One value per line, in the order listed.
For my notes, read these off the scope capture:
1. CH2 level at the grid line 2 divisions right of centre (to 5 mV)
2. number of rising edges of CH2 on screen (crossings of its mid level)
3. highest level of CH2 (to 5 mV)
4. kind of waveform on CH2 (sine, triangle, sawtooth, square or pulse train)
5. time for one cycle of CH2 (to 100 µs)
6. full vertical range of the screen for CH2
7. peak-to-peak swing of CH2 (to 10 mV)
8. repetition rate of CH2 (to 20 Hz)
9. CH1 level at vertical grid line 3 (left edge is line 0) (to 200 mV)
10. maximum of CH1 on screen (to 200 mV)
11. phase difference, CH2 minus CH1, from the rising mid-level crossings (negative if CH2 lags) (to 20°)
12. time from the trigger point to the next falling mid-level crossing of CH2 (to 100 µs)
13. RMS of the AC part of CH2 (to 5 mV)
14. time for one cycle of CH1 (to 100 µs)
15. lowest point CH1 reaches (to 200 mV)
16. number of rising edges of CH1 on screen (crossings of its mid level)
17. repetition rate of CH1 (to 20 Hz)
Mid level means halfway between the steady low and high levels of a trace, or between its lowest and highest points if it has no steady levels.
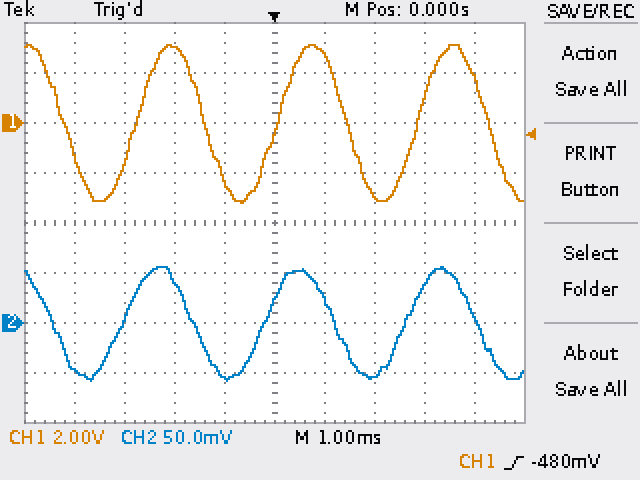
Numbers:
-55 mV
3
55 mV
sine
2.8 ms
400 mV
110 mV
360 Hz
3.0 V
3.2 V
+40°
1.2 ms
40 mV
2.8 ms
-3.2 V
3
360 Hz
